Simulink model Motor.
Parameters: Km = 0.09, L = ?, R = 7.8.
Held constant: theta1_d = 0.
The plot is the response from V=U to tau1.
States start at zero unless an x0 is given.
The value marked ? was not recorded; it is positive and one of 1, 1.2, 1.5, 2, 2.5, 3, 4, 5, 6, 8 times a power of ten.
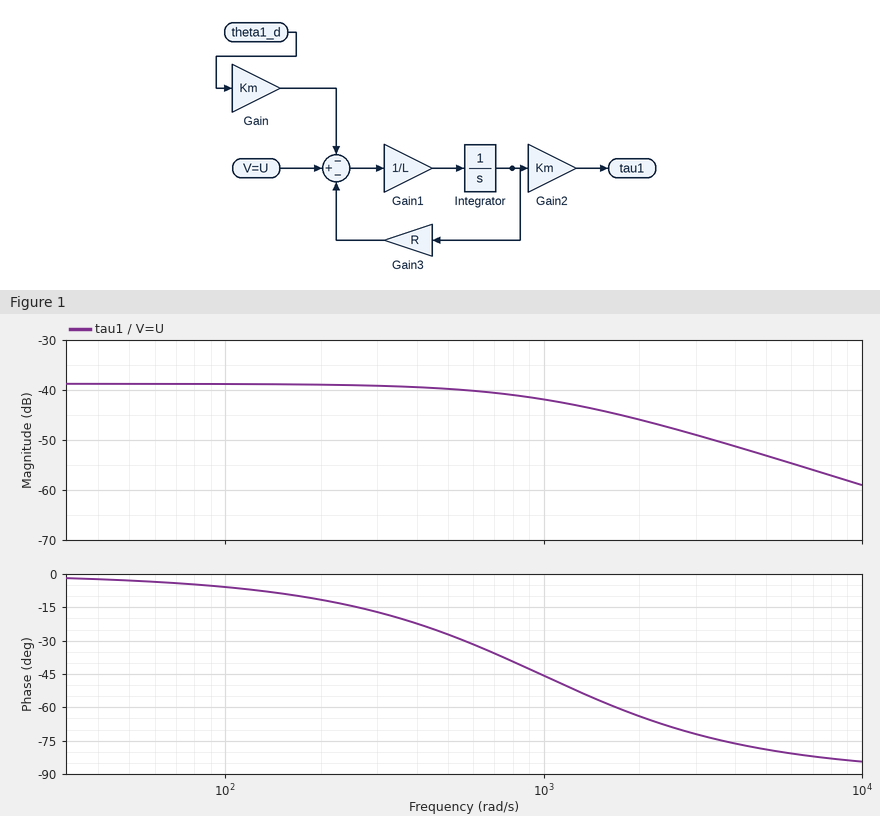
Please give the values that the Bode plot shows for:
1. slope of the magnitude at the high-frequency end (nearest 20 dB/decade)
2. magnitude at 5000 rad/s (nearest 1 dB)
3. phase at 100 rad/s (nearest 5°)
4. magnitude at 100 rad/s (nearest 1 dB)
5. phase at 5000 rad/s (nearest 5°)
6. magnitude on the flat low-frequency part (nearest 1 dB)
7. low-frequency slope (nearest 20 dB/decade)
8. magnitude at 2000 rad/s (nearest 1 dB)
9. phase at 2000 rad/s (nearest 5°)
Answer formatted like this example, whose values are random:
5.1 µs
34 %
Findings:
-20 dB/decade
-53 dB
-5°
-39 dB
-80°
-39 dB
0 dB/decade
-46 dB
-65°
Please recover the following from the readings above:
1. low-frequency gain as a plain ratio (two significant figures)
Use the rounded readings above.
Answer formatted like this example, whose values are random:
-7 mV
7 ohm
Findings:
0.011
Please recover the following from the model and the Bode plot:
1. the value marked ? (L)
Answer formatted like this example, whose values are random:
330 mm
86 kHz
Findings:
0.008
